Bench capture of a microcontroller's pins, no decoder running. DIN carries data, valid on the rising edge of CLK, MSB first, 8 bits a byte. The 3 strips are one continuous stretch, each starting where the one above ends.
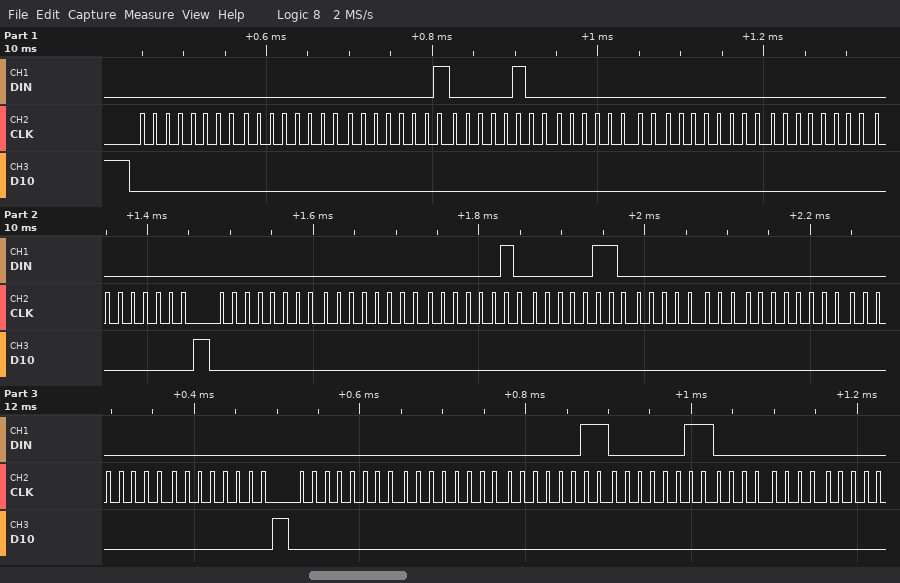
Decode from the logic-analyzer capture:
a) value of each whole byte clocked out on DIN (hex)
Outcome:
00 00 01 04 00 00 00 00 00 00 02 06 00 00 00 00 00 00 03 03 00
